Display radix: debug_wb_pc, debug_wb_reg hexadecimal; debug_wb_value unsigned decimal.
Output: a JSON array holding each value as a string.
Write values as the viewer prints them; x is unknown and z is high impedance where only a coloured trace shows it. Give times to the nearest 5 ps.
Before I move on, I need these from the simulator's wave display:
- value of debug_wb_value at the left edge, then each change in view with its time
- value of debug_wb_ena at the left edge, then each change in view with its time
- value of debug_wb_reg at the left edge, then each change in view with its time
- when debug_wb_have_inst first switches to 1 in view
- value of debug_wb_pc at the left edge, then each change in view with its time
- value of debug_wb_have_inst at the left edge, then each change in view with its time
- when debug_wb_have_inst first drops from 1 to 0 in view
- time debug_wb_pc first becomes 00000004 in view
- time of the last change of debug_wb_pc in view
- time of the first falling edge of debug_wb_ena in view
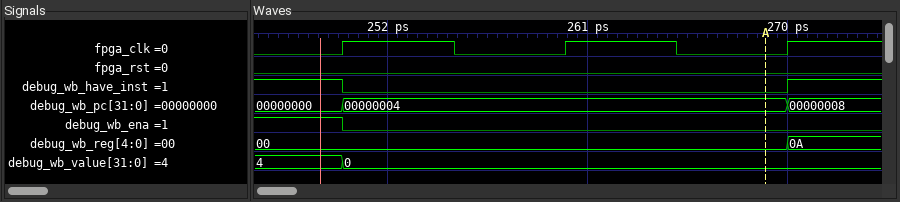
["4, 0 at 250 ps", "1, 0 at 250 ps", "00, 0A at 270 ps", "270 ps", "00000000, 00000004 at 250 ps, 00000008 at 270 ps", "1, 0 at 250 ps, 1 at 270 ps", "250 ps", "250 ps", "270 ps", "250 ps"]
